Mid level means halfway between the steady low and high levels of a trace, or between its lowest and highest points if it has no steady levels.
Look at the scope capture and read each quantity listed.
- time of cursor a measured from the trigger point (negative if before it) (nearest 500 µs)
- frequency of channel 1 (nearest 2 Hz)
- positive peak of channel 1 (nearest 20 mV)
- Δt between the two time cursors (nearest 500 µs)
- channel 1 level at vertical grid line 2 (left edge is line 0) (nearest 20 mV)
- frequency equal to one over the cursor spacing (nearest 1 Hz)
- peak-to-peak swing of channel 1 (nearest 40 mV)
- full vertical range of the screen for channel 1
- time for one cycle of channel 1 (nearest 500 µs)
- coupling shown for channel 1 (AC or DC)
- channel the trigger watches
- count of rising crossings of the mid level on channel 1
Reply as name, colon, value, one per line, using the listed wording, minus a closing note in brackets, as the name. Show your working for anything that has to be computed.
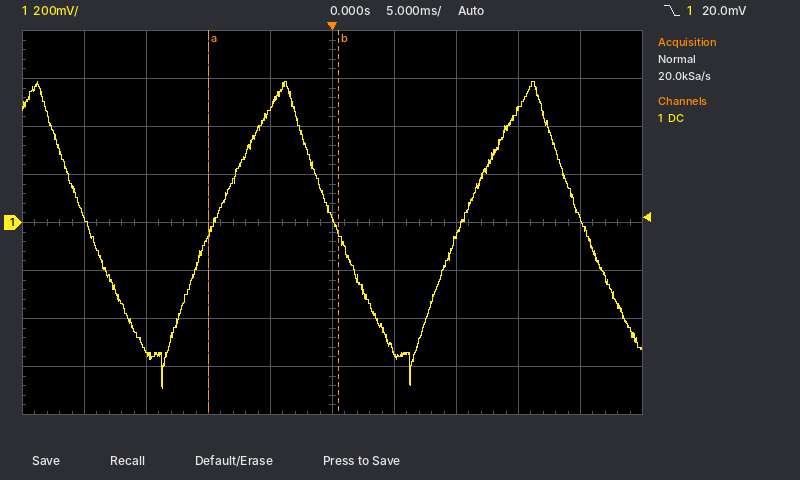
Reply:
time of cursor a measured from the trigger point (negative if before it): -10.0 ms
frequency of channel 1: 1 / 20.0 ms ≈ 50 Hz
positive peak of channel 1: 580 mV
Δt between the two time cursors: 10.5 ms
channel 1 level at vertical grid line 2 (left edge is line 0): -540 mV
frequency equal to one over the cursor spacing: 1 / 10.5 ms ≈ 95 Hz
peak-to-peak swing of channel 1: 1.28 V
full vertical range of the screen for channel 1: 1.6 V
time for one cycle of channel 1: 20.0 ms
coupling shown for channel 1: DC
channel the trigger watches: channel 1
count of rising crossings of the mid level on channel 1: 2
